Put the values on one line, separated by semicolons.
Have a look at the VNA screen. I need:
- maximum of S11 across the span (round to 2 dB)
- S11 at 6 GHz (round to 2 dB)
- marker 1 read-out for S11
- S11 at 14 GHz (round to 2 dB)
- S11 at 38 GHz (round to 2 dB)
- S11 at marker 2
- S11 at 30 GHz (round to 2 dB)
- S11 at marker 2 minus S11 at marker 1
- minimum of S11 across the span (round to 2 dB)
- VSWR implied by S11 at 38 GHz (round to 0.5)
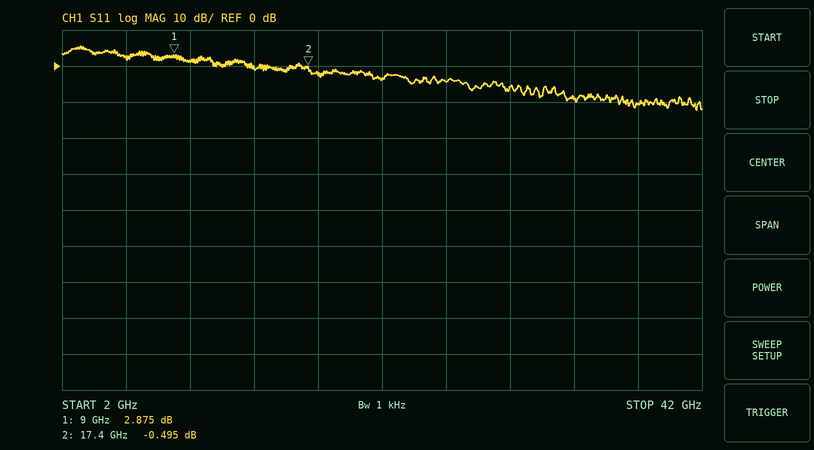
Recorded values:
6 dB; 2 dB; 2.875 dB; 0 dB; -10 dB; -0.495 dB; -6 dB; -3.370 dB; -12 dB; 2.0
